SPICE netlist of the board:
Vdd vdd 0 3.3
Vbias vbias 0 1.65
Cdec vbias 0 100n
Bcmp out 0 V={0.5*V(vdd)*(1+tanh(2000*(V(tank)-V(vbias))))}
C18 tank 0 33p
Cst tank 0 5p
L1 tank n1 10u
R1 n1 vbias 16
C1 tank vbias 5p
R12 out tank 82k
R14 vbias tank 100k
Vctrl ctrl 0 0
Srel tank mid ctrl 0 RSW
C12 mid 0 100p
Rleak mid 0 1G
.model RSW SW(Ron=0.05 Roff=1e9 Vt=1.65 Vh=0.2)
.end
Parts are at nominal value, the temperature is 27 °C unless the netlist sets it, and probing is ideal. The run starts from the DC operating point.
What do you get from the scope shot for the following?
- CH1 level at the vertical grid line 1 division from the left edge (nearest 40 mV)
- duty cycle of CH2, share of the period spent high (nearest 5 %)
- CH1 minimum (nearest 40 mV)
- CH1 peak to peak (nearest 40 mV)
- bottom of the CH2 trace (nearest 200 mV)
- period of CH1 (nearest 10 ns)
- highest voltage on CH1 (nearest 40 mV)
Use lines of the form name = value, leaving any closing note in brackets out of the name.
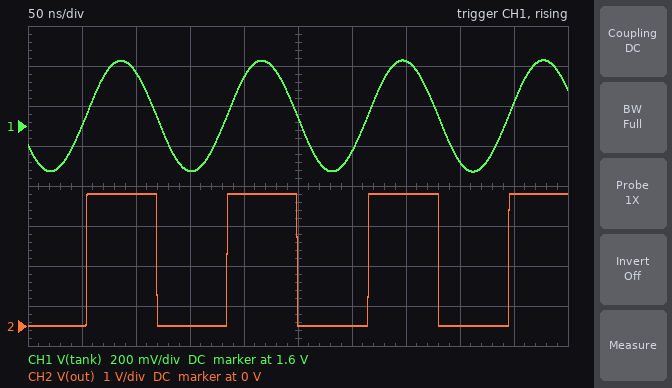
CH1 level at the vertical grid line 1 division from the left edge = 1.60 V
duty cycle of CH2, share of the period spent high = 50 %
CH1 minimum = 1.36 V
CH1 peak to peak = 560 mV
bottom of the CH2 trace = 0 V
period of CH1 = 130 ns
highest voltage on CH1 = 1.92 V
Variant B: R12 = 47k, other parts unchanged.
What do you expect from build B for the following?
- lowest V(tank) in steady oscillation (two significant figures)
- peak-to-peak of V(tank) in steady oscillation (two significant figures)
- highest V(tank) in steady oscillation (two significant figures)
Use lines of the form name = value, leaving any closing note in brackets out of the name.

lowest V(tank) in steady oscillation = 1.2 V
peak-to-peak of V(tank) in steady oscillation = 890 mV
highest V(tank) in steady oscillation = 2.1 V
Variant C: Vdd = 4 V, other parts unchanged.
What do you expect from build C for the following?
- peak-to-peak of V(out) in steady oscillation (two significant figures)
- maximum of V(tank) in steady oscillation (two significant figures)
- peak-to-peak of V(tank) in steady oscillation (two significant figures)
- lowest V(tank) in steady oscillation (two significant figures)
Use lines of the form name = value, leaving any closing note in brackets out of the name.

peak-to-peak of V(out) in steady oscillation = 4.0 V
maximum of V(tank) in steady oscillation = 2.0 V
peak-to-peak of V(tank) in steady oscillation = 680 mV
lowest V(tank) in steady oscillation = 1.3 V
